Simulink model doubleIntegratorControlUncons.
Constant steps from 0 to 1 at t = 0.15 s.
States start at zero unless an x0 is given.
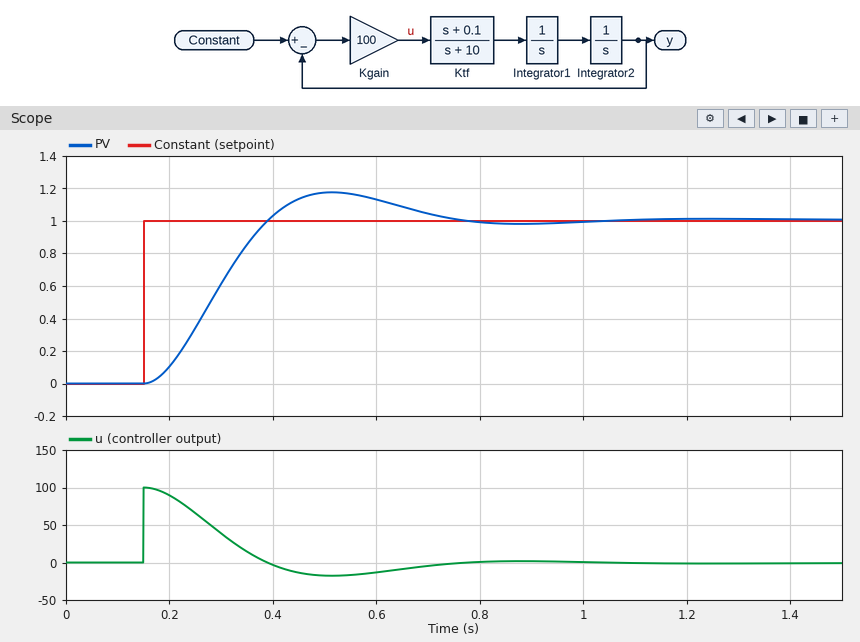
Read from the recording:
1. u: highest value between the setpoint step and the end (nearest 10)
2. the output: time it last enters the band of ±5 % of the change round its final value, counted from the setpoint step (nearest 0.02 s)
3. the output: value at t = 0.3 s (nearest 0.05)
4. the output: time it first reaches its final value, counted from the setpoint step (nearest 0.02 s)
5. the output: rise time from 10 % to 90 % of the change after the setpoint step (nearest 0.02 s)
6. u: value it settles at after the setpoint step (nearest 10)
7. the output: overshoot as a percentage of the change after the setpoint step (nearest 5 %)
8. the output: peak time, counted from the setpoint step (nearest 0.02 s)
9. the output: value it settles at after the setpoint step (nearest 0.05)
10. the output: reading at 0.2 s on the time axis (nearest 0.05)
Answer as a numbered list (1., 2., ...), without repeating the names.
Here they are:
1. 100
2. 0.54 s
3. 0.60
4. 0.24 s
5. 0.16 s
6. 0
7. 15 %
8. 0.36 s
9. 1.00
10. 0.10
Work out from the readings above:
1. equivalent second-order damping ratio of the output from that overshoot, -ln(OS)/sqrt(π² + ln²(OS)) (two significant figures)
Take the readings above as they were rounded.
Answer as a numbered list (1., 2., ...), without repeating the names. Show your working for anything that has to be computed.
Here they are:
1. ln(0.15) = -1.897; 1.897 / sqrt(9.870 + 3.599) = 0.52
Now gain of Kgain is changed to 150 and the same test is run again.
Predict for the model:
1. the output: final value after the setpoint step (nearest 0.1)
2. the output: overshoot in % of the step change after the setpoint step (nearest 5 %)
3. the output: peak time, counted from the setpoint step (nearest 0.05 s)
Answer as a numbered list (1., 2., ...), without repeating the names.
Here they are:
1. 1.0
2. 25 %
3. 0.30 s
